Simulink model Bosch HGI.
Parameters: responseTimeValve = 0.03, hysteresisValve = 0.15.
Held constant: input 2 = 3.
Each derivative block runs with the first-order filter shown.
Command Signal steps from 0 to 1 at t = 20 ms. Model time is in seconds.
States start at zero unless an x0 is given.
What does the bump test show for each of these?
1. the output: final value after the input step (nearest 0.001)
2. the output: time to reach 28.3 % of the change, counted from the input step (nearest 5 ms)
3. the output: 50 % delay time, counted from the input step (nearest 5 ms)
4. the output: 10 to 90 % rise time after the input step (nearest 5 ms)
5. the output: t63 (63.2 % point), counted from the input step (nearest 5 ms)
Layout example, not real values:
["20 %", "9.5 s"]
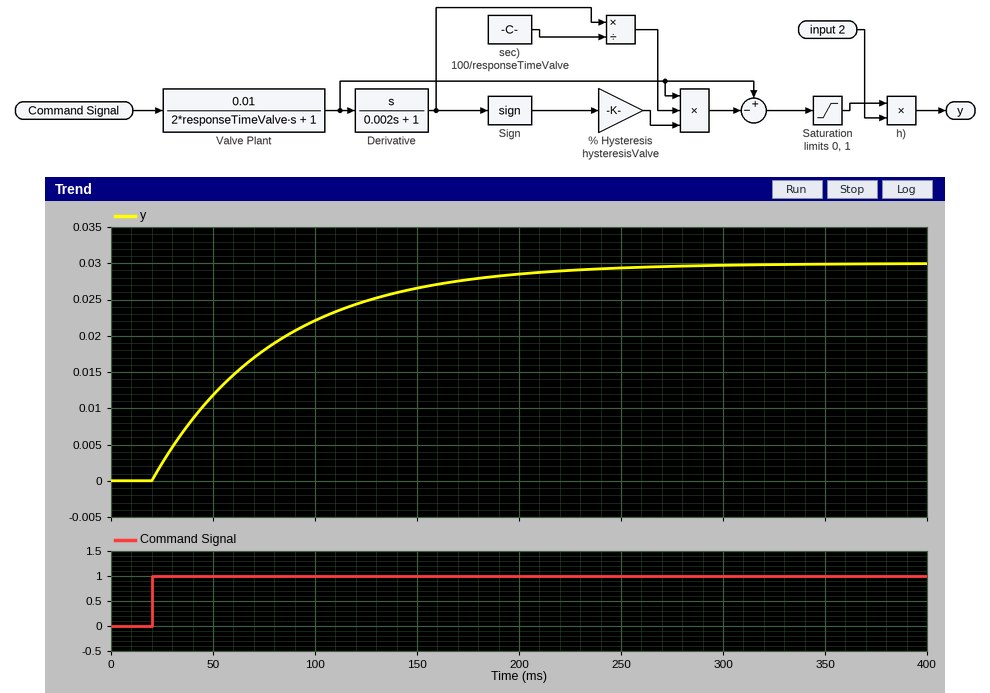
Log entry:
["0.030", "20 ms", "40 ms", "130 ms", "60 ms"]
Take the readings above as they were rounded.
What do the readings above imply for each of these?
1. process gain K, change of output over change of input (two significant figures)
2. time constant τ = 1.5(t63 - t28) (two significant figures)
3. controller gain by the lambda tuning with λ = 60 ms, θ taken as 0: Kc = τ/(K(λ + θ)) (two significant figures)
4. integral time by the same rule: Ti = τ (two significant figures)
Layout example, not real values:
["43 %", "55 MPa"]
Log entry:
["0.030", "60 ms", "33", "60 ms"]
